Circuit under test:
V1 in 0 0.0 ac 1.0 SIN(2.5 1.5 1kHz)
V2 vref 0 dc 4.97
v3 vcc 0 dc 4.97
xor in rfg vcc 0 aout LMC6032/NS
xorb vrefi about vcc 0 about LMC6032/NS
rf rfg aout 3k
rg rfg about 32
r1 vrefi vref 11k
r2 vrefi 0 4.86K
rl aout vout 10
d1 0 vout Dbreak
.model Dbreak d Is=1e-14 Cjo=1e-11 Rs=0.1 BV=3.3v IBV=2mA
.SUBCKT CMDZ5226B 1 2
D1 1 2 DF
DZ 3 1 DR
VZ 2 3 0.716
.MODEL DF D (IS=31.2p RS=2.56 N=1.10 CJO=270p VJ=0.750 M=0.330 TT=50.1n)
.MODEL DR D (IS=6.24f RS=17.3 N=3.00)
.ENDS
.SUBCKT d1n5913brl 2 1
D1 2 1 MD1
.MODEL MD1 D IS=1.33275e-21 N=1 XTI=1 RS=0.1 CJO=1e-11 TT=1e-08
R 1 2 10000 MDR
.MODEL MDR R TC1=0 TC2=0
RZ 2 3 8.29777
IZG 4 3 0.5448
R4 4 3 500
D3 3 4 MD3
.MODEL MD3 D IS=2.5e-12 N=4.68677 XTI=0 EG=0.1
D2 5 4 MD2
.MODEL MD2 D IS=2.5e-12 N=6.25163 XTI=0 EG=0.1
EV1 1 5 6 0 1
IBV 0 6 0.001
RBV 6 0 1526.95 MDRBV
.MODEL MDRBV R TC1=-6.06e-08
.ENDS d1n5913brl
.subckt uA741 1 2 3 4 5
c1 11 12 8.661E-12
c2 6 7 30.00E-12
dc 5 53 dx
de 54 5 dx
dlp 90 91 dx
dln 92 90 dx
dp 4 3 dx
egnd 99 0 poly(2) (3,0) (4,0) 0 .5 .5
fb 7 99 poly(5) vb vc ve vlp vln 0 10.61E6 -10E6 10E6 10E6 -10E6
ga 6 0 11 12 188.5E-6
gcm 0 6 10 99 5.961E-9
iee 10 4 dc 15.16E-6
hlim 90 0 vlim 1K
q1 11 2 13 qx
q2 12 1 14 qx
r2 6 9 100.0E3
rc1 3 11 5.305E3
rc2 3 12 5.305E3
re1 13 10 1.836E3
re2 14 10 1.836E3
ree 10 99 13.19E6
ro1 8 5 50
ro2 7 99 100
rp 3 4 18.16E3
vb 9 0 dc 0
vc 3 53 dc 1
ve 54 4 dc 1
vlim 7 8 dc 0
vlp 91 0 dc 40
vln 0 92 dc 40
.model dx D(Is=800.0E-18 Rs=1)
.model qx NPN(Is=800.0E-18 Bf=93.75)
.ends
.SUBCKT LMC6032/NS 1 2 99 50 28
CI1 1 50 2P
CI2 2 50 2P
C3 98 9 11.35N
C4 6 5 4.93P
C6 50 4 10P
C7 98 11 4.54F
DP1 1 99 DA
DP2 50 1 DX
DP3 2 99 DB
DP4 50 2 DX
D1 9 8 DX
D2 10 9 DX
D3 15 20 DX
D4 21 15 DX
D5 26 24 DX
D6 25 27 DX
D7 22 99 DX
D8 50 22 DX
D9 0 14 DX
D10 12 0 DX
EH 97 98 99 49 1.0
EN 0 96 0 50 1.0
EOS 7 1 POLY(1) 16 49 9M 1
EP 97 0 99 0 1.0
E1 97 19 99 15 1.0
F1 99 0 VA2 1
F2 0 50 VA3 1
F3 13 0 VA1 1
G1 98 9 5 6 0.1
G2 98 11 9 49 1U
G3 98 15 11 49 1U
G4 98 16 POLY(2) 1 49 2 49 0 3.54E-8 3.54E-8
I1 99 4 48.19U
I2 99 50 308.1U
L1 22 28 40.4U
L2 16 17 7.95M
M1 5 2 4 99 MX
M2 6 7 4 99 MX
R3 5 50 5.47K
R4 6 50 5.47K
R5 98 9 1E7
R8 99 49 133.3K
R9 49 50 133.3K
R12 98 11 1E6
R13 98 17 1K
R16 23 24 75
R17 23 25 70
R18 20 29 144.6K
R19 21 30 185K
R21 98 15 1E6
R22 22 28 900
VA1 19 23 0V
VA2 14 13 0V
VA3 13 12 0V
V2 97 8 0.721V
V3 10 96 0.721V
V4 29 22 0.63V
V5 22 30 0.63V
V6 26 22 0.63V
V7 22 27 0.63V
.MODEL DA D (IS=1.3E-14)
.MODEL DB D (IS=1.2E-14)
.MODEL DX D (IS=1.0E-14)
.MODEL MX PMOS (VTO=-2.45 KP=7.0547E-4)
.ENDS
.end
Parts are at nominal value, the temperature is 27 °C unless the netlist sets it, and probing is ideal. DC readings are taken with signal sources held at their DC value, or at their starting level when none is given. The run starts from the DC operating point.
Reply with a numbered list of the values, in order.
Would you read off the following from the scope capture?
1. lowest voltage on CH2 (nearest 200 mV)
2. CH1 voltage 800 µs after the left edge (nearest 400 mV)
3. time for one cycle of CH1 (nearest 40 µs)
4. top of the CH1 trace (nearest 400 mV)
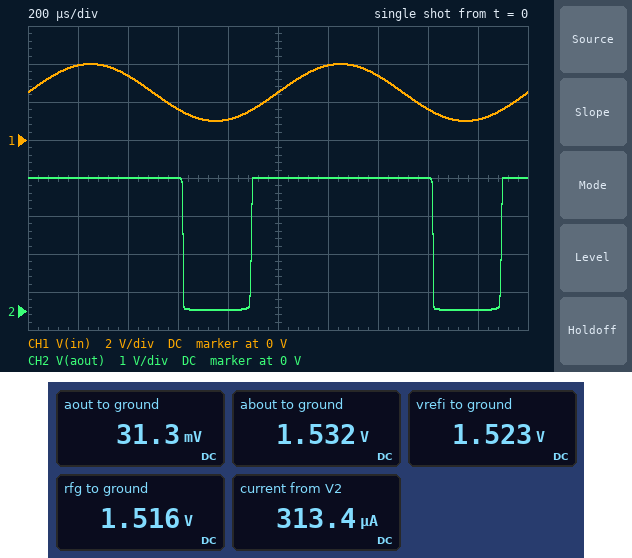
1. 0 V
2. 1.2 V
3. 1.00 ms
4. 4.0 V
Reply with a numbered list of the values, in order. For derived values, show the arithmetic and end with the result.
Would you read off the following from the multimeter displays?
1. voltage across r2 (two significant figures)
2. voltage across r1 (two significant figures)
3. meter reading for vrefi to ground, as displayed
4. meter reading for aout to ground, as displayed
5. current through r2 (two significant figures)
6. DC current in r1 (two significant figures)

1. 1.523 V = 1.5 V
2. 4.97 V - 1.523 V = 3.4 V
3. 1.523 V
4. 31.3 mV
5. (1.523 V) / 4.86 kΩ = 310 µA
6. (4.97 V - 1.523 V) / 11 kΩ = 310 µA
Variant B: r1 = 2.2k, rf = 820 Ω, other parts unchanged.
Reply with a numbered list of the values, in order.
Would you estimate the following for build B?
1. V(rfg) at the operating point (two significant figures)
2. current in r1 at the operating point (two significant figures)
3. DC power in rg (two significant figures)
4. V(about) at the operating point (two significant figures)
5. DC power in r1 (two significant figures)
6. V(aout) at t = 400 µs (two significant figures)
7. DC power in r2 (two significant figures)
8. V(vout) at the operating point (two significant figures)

1. 3.0 V
2. 700 µA
3. 340 µW
4. 3.1 V
5. 1.1 mW
6. 1.2 V
7. 2.4 mW
8. 280 mV
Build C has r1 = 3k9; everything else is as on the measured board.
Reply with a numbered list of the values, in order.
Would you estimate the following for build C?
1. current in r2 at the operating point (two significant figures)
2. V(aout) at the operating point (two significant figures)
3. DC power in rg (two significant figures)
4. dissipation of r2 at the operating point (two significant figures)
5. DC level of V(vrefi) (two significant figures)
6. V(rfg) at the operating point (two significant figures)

1. 570 µA
2. 71 mV
3. 25 µW
4. 1.6 mW
5. 2.8 V
6. 2.7 V
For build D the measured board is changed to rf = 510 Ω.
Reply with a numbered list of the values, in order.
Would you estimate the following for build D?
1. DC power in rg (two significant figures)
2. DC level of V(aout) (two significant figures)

1. 190 µW
2. 210 mV
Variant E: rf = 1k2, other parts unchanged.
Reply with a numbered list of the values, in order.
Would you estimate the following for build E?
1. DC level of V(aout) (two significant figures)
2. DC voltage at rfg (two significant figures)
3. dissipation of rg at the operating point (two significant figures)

1. 98 mV
2. 1.5 V
3. 43 µW
